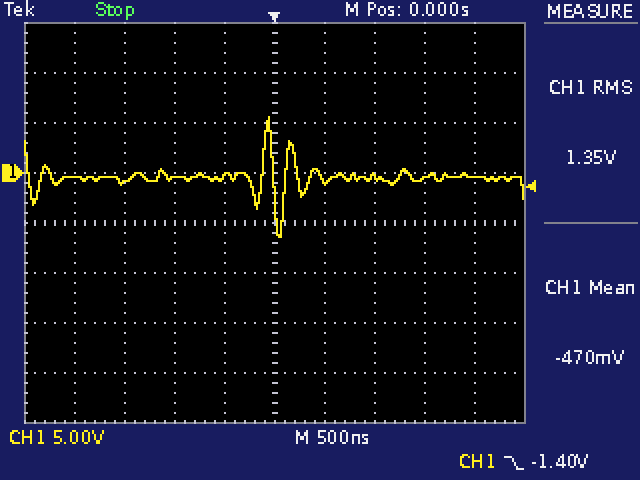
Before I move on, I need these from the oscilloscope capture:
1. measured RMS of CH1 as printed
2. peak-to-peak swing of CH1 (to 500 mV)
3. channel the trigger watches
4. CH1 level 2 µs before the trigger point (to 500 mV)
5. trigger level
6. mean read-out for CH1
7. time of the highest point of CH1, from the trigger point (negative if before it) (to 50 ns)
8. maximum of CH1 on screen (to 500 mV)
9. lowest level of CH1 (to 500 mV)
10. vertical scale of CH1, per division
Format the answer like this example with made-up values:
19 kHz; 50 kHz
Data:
1.35 V; 12.0 V; CH1; -500 mV; -1.40 V; -470 mV; -50 ns; 5.5 V; -6.5 V; 5 V
